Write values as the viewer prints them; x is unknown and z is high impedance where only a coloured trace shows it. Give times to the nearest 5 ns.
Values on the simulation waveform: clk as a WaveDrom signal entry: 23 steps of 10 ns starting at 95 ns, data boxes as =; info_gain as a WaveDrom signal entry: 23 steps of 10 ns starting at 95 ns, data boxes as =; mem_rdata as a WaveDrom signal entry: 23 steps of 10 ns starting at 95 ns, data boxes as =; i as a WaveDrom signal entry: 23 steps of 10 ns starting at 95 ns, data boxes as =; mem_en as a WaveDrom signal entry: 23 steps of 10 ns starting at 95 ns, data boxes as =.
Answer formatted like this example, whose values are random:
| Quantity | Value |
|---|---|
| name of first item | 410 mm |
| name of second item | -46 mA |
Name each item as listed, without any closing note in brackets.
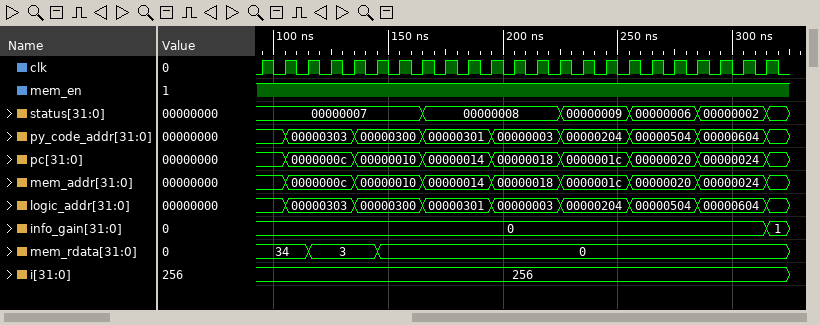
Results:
| Quantity | Value |
|---|---|
| clk as a WaveDrom signal entry: 23 steps of 10 ns starting at 95 ns, data boxes as = | {name: 'clk', wave: 'p......................'} |
| info_gain as a WaveDrom signal entry: 23 steps of 10 ns starting at 95 ns, data boxes as = | {name: 'info_gain', wave: '=.....................=', data: '0 1'} |
| mem_rdata as a WaveDrom signal entry: 23 steps of 10 ns starting at 95 ns, data boxes as = | {name: 'mem_rdata', wave: '=.=..=.................', data: '34 3 0'} |
| i as a WaveDrom signal entry: 23 steps of 10 ns starting at 95 ns, data boxes as = | {name: 'i', wave: '=......................', data: '256'} |
| mem_en as a WaveDrom signal entry: 23 steps of 10 ns starting at 95 ns, data boxes as = | {name: 'mem_en', wave: '1......................'} |
